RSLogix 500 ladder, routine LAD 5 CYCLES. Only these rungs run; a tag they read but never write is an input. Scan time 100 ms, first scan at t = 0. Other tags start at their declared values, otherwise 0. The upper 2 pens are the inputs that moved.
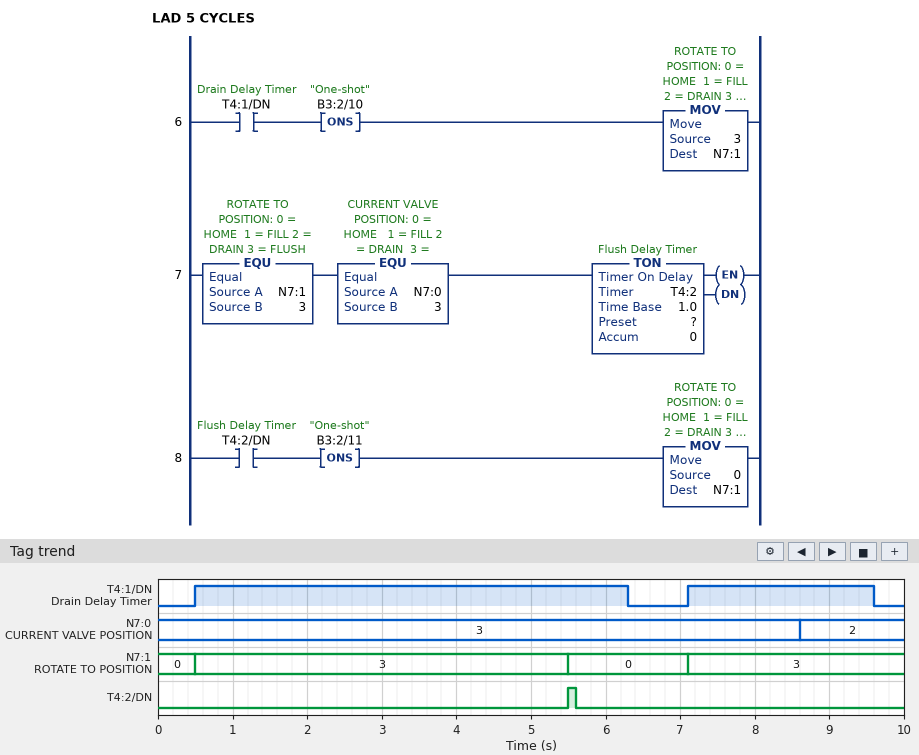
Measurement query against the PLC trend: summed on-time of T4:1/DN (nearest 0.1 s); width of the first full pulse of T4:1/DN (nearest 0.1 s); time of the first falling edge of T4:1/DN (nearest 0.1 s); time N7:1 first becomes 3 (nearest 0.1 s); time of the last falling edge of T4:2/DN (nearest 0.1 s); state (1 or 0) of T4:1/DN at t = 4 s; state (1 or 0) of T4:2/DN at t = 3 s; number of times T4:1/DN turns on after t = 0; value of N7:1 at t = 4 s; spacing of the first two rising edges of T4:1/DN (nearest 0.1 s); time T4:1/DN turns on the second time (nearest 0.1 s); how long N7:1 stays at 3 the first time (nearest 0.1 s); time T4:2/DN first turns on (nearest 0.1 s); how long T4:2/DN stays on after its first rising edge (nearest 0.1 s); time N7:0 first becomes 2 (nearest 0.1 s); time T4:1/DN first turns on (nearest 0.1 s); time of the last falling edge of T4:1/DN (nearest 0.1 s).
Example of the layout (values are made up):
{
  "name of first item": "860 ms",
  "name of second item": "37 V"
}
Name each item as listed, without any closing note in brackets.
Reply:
{
  "summed on-time of T4:1/DN": "8.3 s",
  "width of the first full pulse of T4:1/DN": "5.8 s",
  "time of the first falling edge of T4:1/DN": "6.3 s",
  "time N7:1 first becomes 3": "0.5 s",
  "time of the last falling edge of T4:2/DN": "5.6 s",
  "state (1 or 0) of T4:1/DN at t = 4 s": "1",
  "state (1 or 0) of T4:2/DN at t = 3 s": "0",
  "number of times T4:1/DN turns on after t = 0": "2",
  "value of N7:1 at t = 4 s": "3",
  "spacing of the first two rising edges of T4:1/DN": "6.6 s",
  "time T4:1/DN turns on the second time": "7.1 s",
  "how long N7:1 stays at 3 the first time": "5.0 s",
  "time T4:2/DN first turns on": "5.5 s",
  "how long T4:2/DN stays on after its first rising edge": "0.1 s",
  "time N7:0 first becomes 2": "8.6 s",
  "time T4:1/DN first turns on": "0.5 s",
  "time of the last falling edge of T4:1/DN": "9.6 s"
}
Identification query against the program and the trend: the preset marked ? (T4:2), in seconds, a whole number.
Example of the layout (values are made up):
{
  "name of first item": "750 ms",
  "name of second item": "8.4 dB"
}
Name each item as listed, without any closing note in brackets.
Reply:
{
  "the preset marked ? (T4:2), in seconds, a whole number": "5 s"
}
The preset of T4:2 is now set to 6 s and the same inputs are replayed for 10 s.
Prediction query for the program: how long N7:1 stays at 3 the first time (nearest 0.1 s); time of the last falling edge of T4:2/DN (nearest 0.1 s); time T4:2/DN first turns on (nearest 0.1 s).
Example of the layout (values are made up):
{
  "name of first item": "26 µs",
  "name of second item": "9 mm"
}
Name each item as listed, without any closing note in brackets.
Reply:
{
  "how long N7:1 stays at 3 the first time": "6.0 s",
  "time of the last falling edge of T4:2/DN": "6.6 s",
  "time T4:2/DN first turns on": "6.5 s"
}
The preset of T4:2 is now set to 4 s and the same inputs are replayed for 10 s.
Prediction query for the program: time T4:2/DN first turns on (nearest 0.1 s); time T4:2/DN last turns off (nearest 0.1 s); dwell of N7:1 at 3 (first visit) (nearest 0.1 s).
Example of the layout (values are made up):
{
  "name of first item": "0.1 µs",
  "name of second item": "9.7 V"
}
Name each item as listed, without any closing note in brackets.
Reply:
{
  "time T4:2/DN first turns on": "4.5 s",
  "time T4:2/DN last turns off": "4.6 s",
  "dwell of N7:1 at 3 (first visit)": "4.0 s"
}
